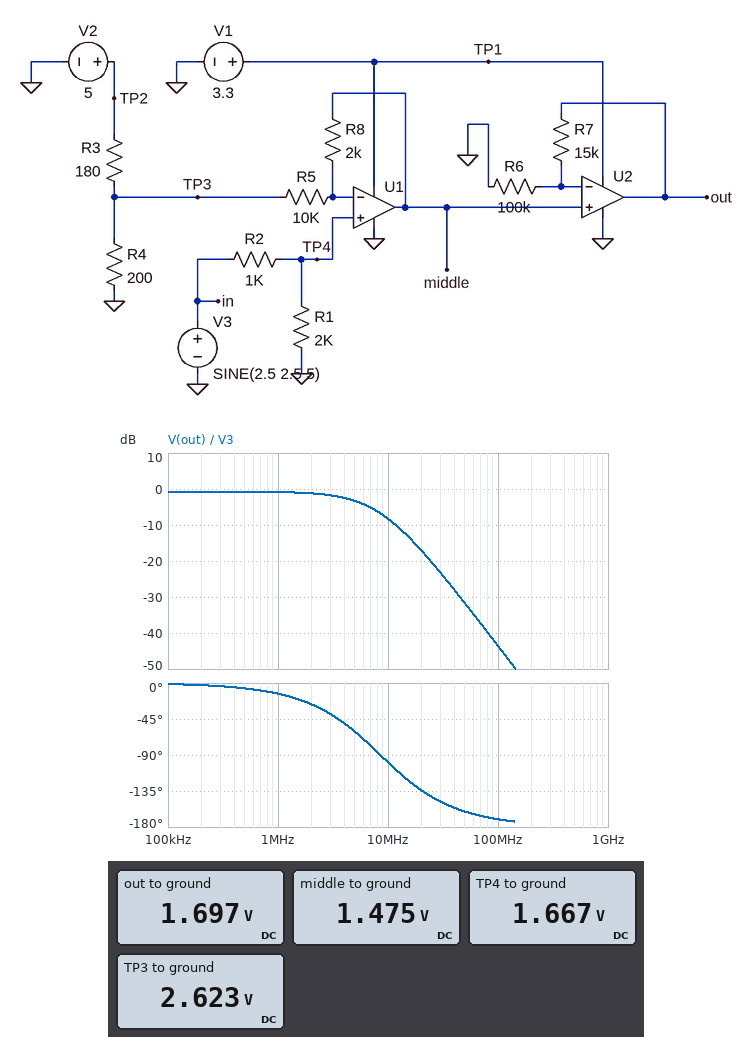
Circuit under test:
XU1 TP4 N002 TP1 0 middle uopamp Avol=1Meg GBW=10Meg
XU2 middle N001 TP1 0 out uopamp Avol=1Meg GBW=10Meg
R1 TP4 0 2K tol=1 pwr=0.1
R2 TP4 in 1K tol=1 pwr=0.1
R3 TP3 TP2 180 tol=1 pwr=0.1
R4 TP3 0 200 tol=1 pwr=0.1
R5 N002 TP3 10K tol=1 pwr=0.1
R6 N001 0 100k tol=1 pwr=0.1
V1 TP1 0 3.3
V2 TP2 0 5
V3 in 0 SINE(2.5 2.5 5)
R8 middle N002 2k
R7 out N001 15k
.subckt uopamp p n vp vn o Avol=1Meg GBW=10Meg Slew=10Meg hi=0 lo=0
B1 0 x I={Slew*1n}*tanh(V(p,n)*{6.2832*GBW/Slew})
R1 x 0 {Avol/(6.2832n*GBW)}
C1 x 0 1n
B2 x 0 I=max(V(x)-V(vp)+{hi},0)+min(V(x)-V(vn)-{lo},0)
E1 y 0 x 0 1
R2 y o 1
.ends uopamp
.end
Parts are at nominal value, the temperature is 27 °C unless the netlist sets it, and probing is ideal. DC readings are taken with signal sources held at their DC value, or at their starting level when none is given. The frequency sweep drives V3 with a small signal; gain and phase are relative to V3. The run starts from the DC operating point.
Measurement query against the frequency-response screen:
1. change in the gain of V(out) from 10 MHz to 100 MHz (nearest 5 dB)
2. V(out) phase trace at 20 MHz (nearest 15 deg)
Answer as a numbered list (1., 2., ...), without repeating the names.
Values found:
1. -35 dB
2. -135 deg
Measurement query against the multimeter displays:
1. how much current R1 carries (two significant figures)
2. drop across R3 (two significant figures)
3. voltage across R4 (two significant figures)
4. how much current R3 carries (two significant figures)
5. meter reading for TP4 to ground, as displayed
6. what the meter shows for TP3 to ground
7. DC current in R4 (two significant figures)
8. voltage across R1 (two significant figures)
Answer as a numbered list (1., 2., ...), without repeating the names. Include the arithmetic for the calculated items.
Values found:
1. (1.667 V) / 2 kΩ = 830 µA
2. 5 V - 2.623 V = 2.4 V
3. 2.623 V = 2.6 V
4. (5 V - 2.623 V) / 180 Ω = 13 mA
5. 1.667 V
6. 2.623 V
7. (2.623 V) / 200 Ω = 13 mA
8. 1.667 V = 1.7 V
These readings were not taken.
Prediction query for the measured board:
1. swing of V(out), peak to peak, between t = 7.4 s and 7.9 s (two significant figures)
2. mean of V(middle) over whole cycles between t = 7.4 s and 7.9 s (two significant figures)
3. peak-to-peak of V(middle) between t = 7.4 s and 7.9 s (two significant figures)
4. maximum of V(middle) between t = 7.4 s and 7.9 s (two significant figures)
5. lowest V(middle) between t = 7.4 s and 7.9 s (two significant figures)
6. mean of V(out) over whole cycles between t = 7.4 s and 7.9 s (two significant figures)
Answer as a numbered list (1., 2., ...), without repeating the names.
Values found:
1. 3.3 V
2. 1.5 V
3. 3.3 V
4. 3.3 V
5. -9.7 mV
6. 1.7 V
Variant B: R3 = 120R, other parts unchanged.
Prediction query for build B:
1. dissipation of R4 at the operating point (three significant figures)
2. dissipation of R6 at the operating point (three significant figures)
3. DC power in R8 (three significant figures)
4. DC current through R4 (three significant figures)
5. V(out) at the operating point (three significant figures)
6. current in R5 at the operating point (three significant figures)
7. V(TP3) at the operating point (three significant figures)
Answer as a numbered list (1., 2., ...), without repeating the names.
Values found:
1. 48.5 mW
2. 19.0 µW
3. 41.9 µW
4. 15.6 mA
5. 1.58 V
6. 145 µA
7. 3.11 V
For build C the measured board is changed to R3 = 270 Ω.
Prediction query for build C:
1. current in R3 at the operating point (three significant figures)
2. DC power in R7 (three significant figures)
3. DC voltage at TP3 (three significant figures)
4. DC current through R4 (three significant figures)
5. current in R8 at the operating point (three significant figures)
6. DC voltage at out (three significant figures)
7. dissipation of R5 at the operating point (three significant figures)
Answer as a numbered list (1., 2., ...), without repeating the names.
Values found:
1. 10.7 mA
2. 3.72 µW
3. 2.12 V
4. 10.6 mA
5. 45.6 µA
6. 1.81 V
7. 20.8 µW
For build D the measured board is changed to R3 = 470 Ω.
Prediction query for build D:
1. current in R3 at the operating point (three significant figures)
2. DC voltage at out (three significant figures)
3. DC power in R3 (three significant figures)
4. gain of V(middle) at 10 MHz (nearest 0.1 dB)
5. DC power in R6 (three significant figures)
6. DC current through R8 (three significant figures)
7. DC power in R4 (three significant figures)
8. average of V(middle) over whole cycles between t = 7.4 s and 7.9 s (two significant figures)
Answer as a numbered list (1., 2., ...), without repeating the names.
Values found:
1. 7.46 mA
2. 1.96 V
3. 26.1 mW
4. -5.8 dB
5. 28.9 µW
6. 17.2 µA
7. 11.2 mW
8. 1.7 V
